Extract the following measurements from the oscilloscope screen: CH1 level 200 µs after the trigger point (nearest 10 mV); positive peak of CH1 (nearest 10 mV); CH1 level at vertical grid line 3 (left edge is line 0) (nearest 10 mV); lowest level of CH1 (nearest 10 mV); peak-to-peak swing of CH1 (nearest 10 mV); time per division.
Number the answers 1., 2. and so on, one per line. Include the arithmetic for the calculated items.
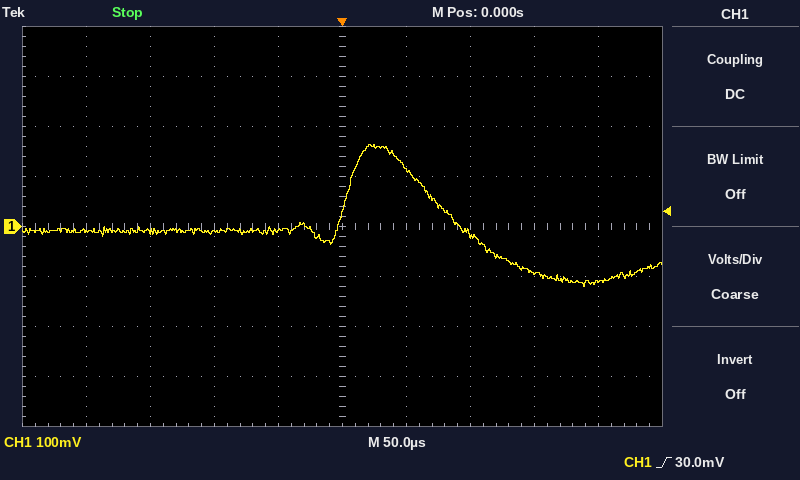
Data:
1. -110 mV
2. 160 mV
3. -10 mV
4. -120 mV
5. 160 mV − (-120 mV) = 280 mV
6. 50 µs
